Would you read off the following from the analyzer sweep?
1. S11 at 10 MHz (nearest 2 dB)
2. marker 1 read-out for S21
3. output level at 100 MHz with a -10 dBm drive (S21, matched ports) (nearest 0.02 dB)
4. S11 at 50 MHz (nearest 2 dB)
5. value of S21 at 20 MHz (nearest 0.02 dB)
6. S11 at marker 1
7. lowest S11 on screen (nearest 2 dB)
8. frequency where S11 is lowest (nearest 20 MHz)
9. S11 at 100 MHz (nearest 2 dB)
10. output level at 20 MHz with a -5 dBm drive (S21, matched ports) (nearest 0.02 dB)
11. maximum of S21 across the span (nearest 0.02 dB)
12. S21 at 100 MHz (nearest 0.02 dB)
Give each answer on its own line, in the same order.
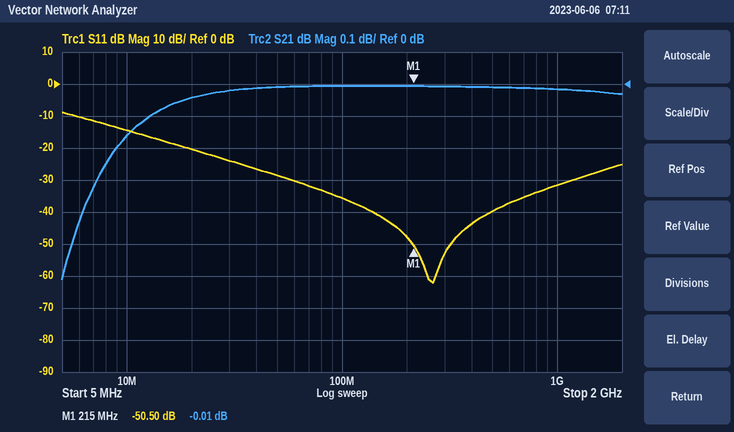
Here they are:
-14 dB
-0.01 dB
-10.00 dBm
-28 dB
-0.04 dB
-50.50 dB
-62 dB
260 MHz
-36 dB
-5.04 dBm
0.00 dB
0.00 dB
